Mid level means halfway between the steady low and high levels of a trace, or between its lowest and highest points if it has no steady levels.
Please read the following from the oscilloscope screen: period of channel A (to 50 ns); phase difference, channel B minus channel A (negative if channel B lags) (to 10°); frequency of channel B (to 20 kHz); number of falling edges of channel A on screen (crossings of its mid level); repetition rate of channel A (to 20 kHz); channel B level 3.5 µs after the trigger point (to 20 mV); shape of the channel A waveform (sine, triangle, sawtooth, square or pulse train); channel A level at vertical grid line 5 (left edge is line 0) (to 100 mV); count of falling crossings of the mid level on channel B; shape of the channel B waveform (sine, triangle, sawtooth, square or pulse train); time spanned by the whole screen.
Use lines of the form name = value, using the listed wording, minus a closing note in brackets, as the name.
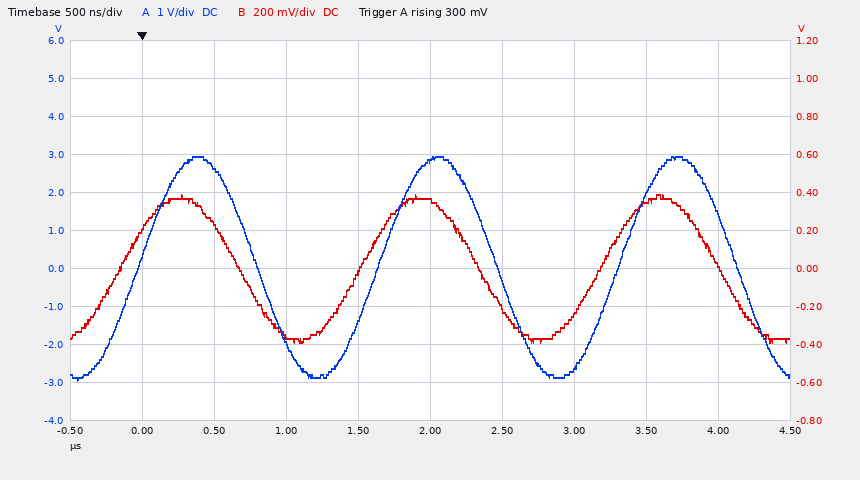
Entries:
period of channel A = 1.65 µs
phase difference, channel B minus channel A (negative if channel B lags) = +30°
frequency of channel B = 600 kHz
number of falling edges of channel A on screen = 3
repetition rate of channel A = 600 kHz
channel B level 3.5 µs after the trigger point = 360 mV
shape of the channel A waveform = sine
channel A level at vertical grid line 5 (left edge is line 0) = 2.9 V
count of falling crossings of the mid level on channel B = 3
shape of the channel B waveform = sine
time spanned by the whole screen = 5 µs
